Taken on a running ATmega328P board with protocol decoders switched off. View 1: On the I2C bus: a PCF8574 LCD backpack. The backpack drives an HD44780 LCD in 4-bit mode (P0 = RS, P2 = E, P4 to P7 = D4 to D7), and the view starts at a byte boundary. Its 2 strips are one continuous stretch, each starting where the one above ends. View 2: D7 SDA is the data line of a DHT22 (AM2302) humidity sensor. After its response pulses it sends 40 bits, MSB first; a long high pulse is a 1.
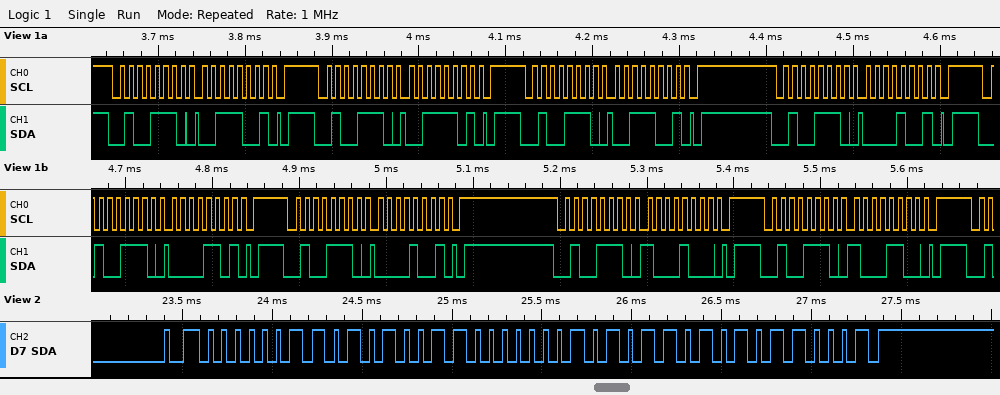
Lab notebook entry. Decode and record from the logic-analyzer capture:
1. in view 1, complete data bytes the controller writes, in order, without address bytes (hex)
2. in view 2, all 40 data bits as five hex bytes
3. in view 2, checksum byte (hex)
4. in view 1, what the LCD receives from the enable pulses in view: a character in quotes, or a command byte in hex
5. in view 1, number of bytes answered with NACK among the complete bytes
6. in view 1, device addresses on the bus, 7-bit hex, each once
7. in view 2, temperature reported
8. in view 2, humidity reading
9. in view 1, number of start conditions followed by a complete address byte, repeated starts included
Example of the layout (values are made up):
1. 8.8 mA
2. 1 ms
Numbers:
1. 39 3D 39 09 0D 09 88 8C
2. 03 53 01 5A B1
3. 0xB1
4. '0'
5. 0
6. 0x27
7. 34.6 °C
8. 85.1 %
9. 8
